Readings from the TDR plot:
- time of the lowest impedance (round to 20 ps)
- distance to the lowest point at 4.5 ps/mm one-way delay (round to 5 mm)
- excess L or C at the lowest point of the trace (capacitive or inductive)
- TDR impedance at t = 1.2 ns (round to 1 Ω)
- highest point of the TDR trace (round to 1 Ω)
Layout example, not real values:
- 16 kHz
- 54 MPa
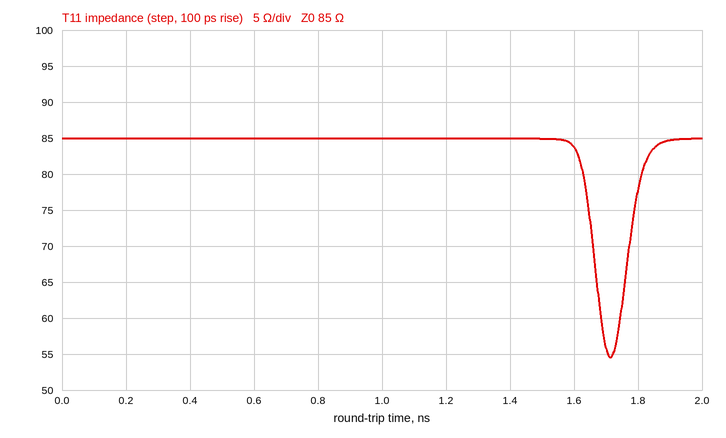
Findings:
- 1.72 ns
- 190 mm
- capacitive
- 85 Ω
- 85 Ω
